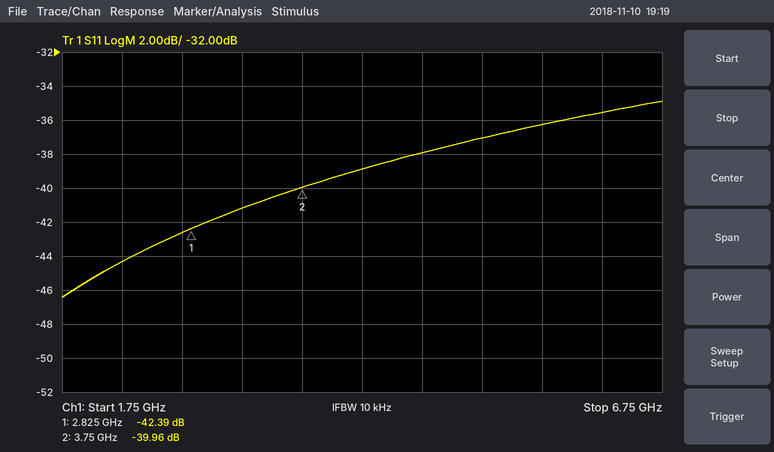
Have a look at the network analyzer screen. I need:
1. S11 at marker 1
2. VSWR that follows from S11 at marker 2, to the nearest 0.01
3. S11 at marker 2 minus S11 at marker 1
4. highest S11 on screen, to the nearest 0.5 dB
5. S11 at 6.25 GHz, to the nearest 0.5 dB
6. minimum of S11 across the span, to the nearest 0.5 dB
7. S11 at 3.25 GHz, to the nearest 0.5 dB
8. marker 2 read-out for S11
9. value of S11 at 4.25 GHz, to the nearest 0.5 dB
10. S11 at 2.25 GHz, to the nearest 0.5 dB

-42.39 dB
1.02
2.43 dB
-35.0 dB
-35.5 dB
-46.5 dB
-41.0 dB
-39.96 dB
-39.0 dB
-44.5 dB
